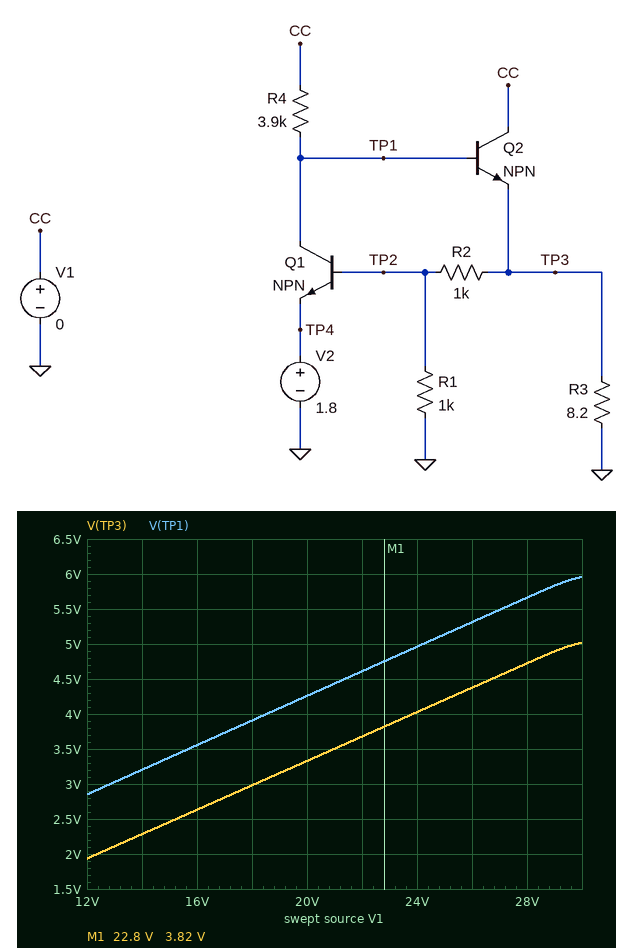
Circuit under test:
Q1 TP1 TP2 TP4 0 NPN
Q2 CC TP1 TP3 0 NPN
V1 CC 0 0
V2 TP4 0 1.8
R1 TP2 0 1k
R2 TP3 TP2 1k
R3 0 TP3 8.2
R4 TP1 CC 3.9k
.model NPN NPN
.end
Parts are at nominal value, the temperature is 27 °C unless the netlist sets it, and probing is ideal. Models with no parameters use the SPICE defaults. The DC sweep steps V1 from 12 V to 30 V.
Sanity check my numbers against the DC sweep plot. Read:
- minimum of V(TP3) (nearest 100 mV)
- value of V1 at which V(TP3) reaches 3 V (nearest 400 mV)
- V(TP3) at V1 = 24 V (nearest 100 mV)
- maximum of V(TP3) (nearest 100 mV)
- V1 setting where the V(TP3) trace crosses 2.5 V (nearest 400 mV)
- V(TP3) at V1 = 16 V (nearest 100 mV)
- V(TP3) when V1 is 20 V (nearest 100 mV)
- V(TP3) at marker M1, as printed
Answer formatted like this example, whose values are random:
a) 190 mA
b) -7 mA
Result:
a) 1.9 V
b) 18.0 V
c) 4.0 V
d) 5.0 V
e) 15.2 V
f) 2.6 V
g) 3.3 V
h) 3.82 V
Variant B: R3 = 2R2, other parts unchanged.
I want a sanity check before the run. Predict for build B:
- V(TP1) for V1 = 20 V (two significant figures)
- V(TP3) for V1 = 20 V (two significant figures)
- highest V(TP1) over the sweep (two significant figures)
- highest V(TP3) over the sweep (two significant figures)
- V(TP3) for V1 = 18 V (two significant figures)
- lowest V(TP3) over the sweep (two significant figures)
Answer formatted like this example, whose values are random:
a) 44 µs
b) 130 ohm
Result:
a) 2.0 V
b) 1.0 V
c) 2.5 V
d) 1.6 V
e) 920 mV
f) 600 mV
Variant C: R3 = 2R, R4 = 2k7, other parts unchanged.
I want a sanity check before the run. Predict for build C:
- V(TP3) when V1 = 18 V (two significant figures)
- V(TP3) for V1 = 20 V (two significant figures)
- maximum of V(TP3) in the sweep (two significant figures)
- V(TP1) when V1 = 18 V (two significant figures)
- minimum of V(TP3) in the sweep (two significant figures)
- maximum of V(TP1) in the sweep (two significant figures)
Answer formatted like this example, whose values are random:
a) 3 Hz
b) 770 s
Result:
a) 1.2 V
b) 1.3 V
c) 2.0 V
d) 2.1 V
e) 770 mV
f) 3.0 V
